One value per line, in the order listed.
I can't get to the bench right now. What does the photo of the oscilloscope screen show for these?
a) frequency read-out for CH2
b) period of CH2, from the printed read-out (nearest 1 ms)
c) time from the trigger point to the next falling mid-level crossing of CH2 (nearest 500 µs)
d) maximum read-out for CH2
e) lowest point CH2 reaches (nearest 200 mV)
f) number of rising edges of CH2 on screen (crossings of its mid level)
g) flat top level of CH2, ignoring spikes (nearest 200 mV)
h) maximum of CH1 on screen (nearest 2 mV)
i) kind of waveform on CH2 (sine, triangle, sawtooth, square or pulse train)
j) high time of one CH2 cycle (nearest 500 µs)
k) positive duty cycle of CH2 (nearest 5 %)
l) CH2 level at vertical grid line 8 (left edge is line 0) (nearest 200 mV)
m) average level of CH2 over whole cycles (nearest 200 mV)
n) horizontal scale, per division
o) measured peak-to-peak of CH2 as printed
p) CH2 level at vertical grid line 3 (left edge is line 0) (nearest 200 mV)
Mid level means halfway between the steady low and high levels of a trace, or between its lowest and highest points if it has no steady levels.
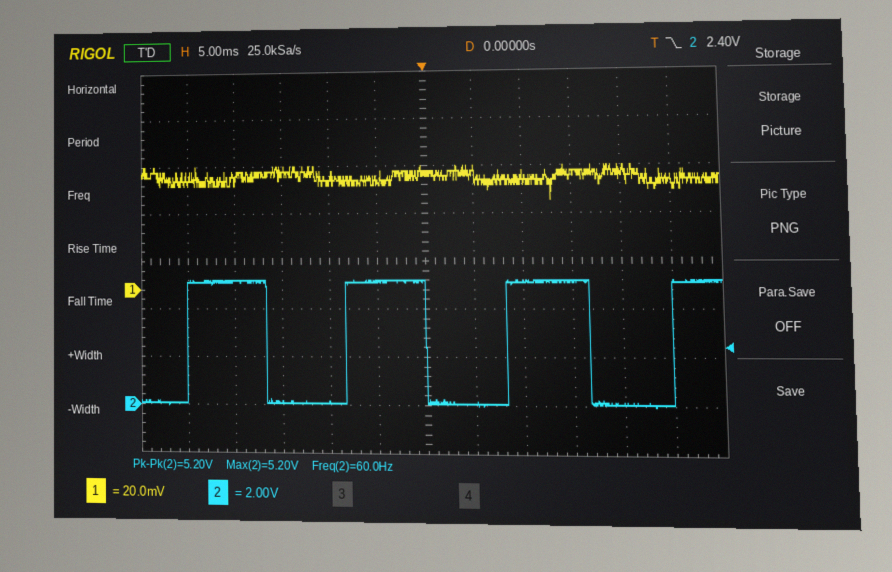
60.0 Hz
17 ms
16.5 ms
5.20 V
0.0 V
4
5.2 V
52 mV
square
8.5 ms
50 %
5.2 V
2.6 V
5 ms
5.20 V
200 mV
